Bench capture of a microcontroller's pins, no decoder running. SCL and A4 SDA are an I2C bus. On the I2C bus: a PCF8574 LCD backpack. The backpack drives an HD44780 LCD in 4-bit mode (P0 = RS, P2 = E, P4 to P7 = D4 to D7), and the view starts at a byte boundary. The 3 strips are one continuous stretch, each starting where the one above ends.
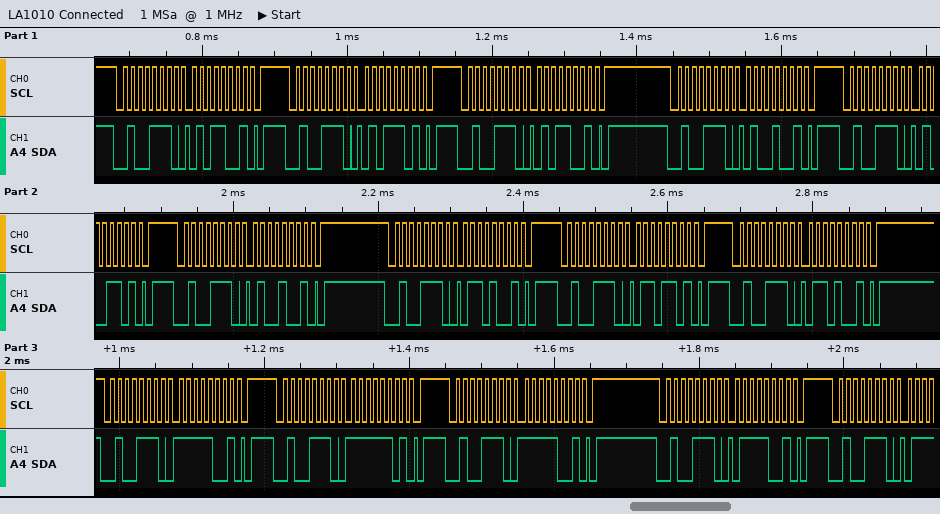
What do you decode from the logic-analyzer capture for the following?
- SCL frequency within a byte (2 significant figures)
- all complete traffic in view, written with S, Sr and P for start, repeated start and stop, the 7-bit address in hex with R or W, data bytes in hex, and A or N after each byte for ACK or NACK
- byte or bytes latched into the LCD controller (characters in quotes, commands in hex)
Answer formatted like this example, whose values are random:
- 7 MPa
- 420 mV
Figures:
- 100 kHz
- S 27W A 59 A P S 27W A 5D A P S 27W A 59 A P S 27W A 49 A P S 27W A 4D A P S 27W A 49 A P S 27W A 69 A P S 27W A 6D A P S 27W A 69 A P S 27W A F9 A P S 27W A FD A P S 27W A F9 A P S 27W A 79 A P S 27W A
- 'T' 'o'
